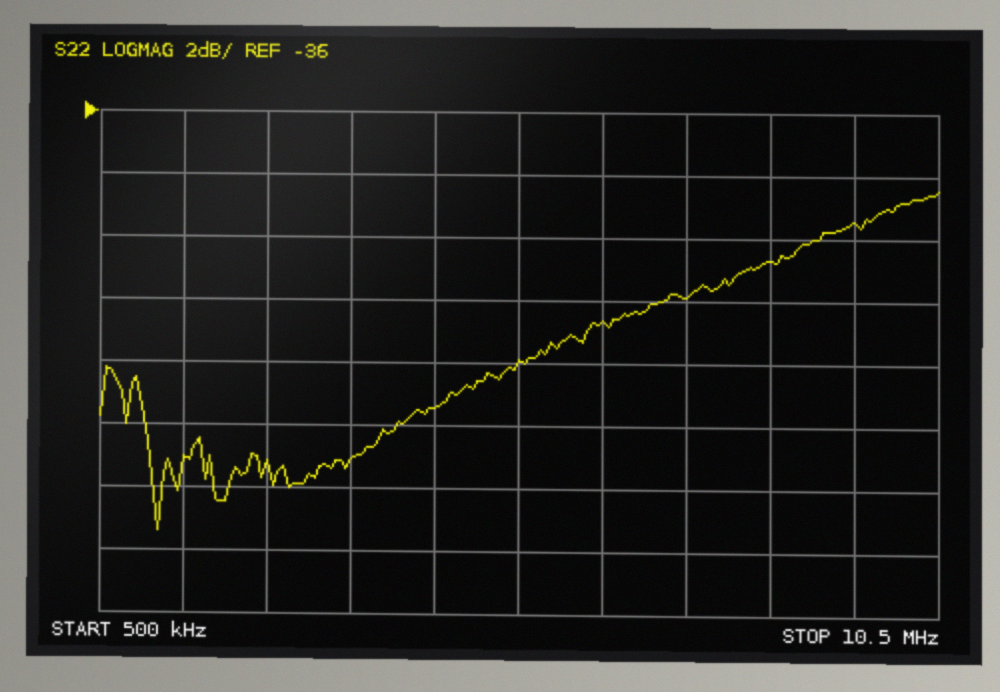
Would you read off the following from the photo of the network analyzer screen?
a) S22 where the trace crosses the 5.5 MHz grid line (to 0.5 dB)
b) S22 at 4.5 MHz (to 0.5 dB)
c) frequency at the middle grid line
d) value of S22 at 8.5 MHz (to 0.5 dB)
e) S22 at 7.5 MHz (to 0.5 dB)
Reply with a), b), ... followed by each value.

a) -44.0 dB
b) -45.5 dB
c) 5.5 MHz
d) -40.5 dB
e) -42.0 dB
